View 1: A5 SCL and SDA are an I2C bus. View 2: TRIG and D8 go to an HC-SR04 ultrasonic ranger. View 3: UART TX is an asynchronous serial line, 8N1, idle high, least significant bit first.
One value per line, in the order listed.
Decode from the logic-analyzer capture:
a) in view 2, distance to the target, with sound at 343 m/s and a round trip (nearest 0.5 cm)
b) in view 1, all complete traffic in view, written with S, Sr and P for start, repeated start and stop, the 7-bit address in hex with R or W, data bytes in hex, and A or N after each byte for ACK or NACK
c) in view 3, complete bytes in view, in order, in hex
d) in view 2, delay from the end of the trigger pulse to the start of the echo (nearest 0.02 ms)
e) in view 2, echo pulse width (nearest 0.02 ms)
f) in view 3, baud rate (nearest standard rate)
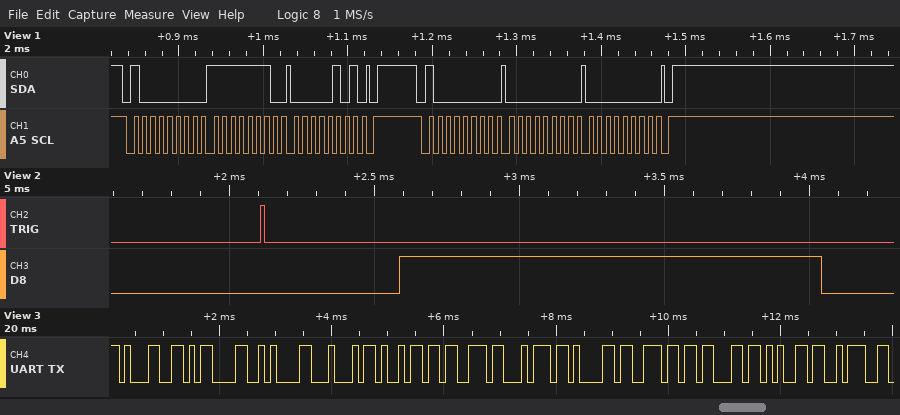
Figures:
25 cm
S 40W A FE A 05 A P S 40W A 00 A 00 A P
31 0D 0A 44 69 73 74 61 6E 63 65 3A
0.46 ms
1.46 ms
9600 baud
